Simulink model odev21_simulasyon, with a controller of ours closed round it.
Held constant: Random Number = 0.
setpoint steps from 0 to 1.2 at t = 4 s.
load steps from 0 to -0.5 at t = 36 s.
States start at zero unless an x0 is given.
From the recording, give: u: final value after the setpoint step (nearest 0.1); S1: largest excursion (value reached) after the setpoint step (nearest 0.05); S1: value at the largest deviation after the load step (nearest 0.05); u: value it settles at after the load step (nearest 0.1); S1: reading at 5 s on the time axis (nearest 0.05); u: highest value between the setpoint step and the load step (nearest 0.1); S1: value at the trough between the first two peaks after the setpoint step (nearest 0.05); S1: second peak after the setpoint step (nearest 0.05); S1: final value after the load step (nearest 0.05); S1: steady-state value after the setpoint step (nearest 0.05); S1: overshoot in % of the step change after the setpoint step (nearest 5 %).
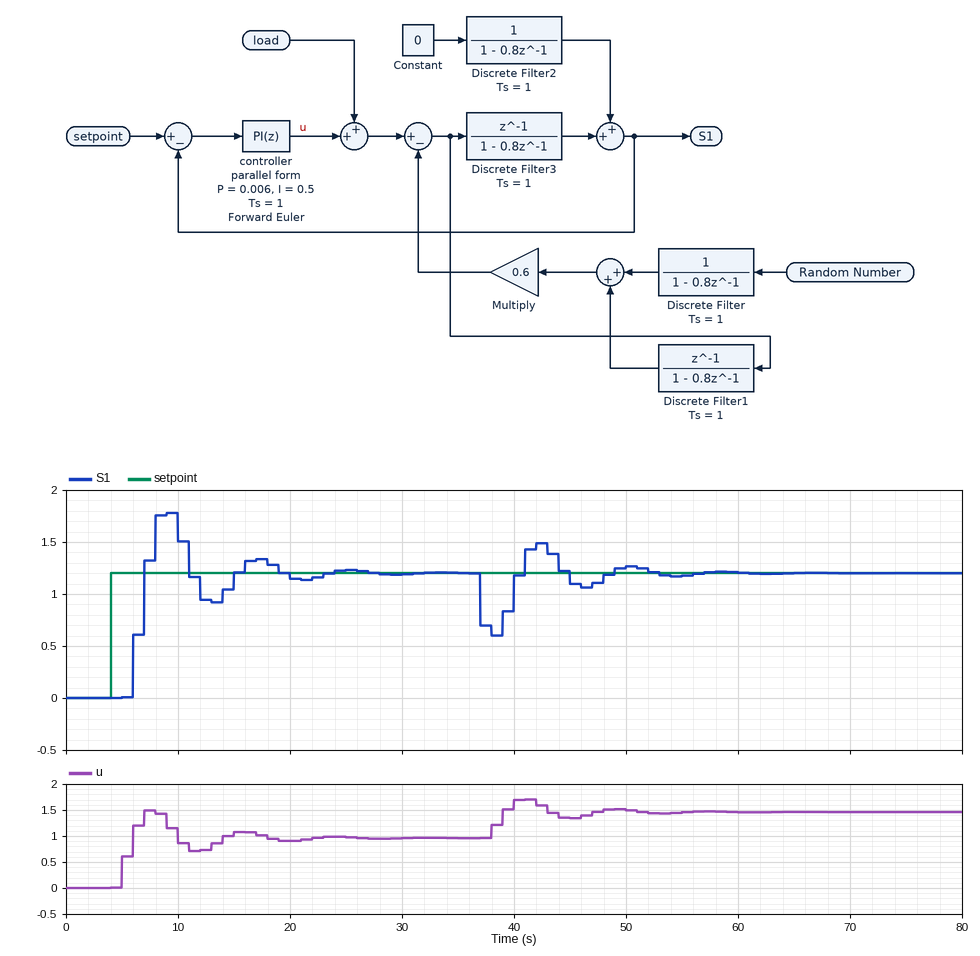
1.0
1.80
0.60
1.5
0.00
1.5
0.90
1.35
1.20
1.20
50 %
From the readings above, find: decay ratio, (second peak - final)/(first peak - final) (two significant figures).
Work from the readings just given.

0.25
